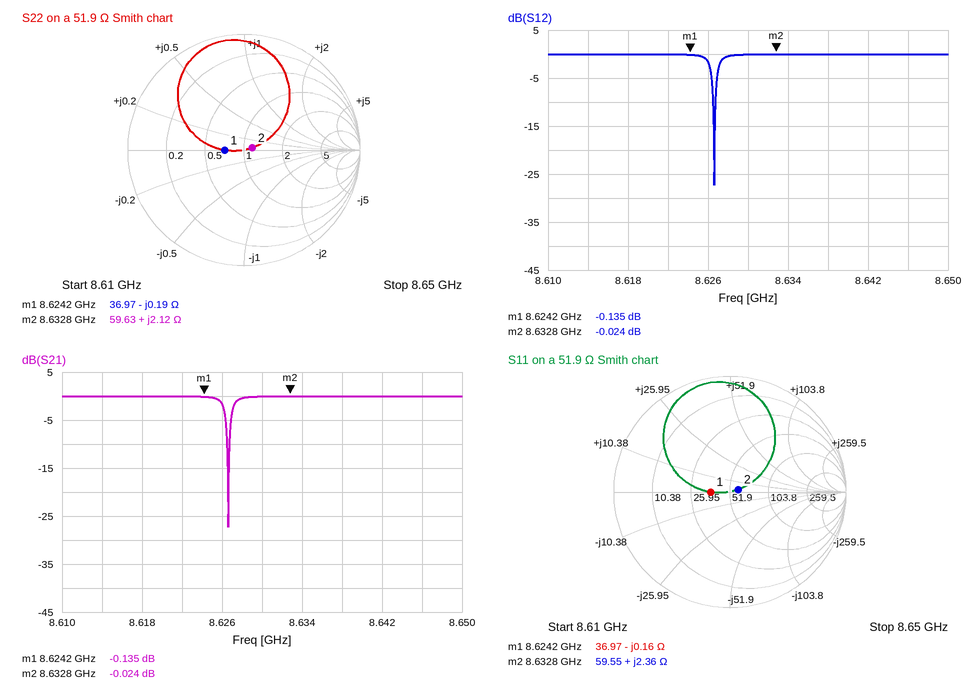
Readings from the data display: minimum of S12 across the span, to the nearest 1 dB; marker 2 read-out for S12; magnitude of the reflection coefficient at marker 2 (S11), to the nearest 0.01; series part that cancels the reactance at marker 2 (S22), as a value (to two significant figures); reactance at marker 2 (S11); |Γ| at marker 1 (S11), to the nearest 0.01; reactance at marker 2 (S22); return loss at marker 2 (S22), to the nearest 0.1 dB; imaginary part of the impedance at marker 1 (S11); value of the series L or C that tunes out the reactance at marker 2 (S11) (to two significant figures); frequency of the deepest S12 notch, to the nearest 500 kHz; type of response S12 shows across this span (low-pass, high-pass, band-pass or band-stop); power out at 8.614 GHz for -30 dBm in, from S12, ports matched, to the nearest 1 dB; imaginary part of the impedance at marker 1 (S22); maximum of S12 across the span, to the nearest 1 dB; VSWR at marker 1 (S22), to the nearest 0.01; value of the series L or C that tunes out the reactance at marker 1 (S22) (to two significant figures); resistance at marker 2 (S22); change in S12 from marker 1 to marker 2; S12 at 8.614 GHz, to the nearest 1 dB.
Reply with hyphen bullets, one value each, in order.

- -27 dB
- -0.024 dB
- 0.07
- 8.7 pF
- +2.36 Ω
- 0.17
- +2.12 Ω
- 22.9 dB
- -0.16 Ω
- 7.8 pF
- 8.6265 GHz
- band-stop
- -30 dBm
- -0.19 Ω
- 0 dB
- 1.40
- 3.5 pH
- 59.63 Ω
- 0.111 dB
- 0 dB
